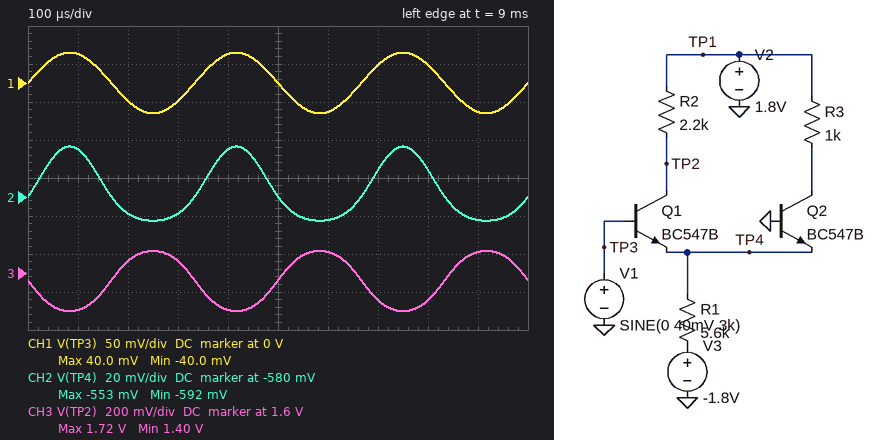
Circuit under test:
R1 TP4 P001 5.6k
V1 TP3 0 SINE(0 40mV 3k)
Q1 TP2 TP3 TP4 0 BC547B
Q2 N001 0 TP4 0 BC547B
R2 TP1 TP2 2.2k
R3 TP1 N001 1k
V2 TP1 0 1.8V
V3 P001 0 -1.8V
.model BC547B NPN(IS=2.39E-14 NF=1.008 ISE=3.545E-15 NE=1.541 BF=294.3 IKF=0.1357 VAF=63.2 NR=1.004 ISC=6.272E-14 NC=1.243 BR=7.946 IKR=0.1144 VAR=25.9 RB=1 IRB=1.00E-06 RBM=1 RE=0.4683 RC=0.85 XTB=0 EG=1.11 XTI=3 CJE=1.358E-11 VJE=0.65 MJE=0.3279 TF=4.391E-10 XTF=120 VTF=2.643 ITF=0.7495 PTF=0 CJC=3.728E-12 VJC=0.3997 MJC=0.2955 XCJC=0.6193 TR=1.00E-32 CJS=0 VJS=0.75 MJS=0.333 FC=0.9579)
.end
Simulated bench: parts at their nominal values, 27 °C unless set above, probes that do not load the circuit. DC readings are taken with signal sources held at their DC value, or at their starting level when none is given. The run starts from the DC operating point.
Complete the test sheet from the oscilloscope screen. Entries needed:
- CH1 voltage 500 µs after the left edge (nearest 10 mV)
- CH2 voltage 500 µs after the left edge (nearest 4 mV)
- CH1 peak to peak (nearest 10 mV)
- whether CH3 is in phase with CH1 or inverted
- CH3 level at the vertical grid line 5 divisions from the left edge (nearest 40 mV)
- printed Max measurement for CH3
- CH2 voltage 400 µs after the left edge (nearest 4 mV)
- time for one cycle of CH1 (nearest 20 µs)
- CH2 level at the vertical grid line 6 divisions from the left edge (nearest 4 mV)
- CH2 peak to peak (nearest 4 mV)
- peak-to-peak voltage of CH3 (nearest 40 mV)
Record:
0 V
-580 mV
80 mV
inverted
1.56 V
1.72 V
-556 mV
340 µs
-592 mV
40 mV
320 mV
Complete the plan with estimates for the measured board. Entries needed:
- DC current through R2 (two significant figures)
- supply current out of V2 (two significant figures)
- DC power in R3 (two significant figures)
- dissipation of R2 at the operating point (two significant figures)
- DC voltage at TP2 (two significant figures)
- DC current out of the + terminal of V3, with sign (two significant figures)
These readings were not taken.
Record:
110 µA
220 µA
12 µW
26 µW
1.6 V
-220 µA
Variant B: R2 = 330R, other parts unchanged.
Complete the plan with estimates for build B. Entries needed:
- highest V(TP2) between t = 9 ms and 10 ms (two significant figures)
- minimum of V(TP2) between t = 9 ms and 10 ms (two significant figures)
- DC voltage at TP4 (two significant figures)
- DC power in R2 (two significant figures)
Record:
1.8 V
1.7 V
-580 mV
3.9 µW
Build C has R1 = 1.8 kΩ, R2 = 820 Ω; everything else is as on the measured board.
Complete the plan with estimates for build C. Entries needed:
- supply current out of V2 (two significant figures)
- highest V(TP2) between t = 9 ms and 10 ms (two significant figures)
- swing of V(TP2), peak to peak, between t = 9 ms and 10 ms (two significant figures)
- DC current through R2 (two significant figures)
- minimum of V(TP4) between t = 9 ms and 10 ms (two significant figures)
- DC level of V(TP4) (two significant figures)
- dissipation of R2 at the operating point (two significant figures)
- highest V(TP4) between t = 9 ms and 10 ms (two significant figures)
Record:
660 µA
1.7 V
360 mV
330 µA
-620 mV
-610 mV
89 µW
-580 mV
